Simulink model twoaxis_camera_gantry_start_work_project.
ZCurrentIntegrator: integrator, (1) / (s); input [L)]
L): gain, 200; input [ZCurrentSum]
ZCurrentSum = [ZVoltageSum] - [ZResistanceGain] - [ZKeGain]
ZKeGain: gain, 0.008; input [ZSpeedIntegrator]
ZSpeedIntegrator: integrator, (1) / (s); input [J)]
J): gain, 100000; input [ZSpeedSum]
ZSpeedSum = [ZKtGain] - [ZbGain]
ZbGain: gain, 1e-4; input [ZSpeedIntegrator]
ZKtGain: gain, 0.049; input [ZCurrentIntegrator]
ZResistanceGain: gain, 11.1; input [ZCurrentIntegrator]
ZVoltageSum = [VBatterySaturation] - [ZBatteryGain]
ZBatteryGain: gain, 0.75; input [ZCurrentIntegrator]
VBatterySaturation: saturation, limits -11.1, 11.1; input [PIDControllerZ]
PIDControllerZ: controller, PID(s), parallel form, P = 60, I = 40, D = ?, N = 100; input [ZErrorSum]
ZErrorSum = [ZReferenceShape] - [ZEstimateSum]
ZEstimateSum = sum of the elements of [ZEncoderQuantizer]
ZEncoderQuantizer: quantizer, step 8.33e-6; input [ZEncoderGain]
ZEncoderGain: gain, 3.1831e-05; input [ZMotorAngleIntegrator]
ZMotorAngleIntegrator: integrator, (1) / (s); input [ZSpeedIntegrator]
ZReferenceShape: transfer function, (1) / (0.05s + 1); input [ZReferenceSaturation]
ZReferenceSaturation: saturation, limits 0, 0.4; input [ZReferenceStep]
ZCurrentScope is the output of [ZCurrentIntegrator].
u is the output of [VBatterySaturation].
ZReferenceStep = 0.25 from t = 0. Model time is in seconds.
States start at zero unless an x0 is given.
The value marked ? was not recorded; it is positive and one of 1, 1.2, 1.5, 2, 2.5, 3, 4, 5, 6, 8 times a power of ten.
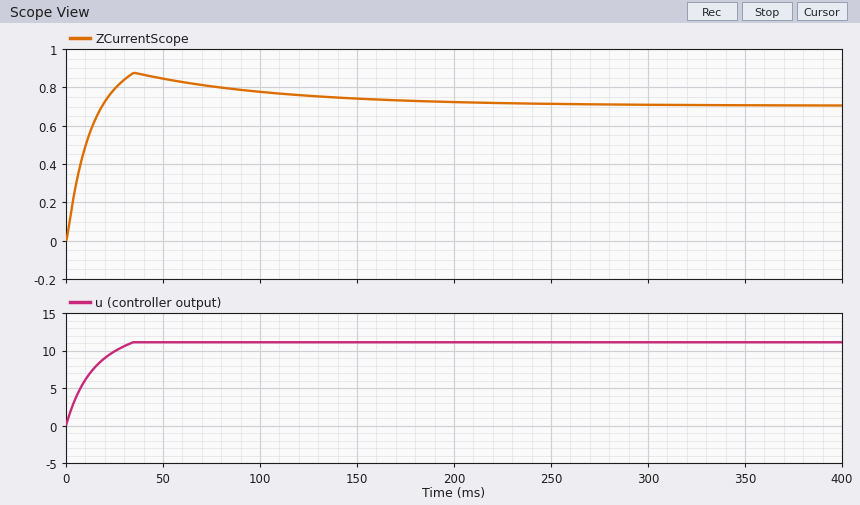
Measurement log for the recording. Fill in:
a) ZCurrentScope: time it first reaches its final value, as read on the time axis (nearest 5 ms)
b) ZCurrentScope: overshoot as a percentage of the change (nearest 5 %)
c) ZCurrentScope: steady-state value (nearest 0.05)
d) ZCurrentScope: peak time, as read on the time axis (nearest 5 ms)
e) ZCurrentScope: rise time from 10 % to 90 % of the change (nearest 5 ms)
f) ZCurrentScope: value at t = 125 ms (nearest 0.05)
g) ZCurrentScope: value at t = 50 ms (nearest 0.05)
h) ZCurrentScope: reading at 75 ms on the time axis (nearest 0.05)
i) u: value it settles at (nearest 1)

20 ms
25 %
0.70
35 ms
15 ms
0.75
0.85
0.80
11
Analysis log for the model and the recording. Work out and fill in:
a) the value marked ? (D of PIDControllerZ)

1.2
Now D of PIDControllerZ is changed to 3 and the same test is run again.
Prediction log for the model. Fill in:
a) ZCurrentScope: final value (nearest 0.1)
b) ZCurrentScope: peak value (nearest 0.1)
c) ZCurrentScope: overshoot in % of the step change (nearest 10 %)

0.7
0.9
30 %
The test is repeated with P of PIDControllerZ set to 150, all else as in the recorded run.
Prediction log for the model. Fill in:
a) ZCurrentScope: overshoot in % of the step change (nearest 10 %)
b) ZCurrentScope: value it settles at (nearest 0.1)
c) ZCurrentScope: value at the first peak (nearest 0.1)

30 %
0.7
0.9
